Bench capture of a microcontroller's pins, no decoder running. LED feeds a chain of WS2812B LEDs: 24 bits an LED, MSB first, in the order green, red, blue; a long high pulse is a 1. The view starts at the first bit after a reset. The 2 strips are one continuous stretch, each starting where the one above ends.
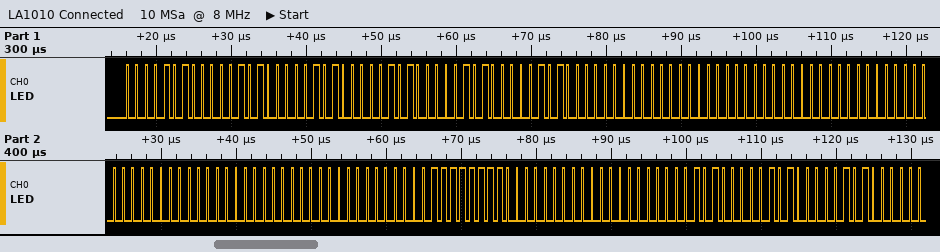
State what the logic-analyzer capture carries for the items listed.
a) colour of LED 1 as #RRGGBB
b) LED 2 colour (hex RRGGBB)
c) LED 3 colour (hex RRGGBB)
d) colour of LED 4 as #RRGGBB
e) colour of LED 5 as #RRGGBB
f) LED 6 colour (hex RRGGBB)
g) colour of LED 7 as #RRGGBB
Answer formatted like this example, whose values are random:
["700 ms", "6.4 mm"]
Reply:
["#0A0A0A", "#0A0A0A", "#000000", "#000000", "#000000", "#00FF00", "#0A0A0A"]
